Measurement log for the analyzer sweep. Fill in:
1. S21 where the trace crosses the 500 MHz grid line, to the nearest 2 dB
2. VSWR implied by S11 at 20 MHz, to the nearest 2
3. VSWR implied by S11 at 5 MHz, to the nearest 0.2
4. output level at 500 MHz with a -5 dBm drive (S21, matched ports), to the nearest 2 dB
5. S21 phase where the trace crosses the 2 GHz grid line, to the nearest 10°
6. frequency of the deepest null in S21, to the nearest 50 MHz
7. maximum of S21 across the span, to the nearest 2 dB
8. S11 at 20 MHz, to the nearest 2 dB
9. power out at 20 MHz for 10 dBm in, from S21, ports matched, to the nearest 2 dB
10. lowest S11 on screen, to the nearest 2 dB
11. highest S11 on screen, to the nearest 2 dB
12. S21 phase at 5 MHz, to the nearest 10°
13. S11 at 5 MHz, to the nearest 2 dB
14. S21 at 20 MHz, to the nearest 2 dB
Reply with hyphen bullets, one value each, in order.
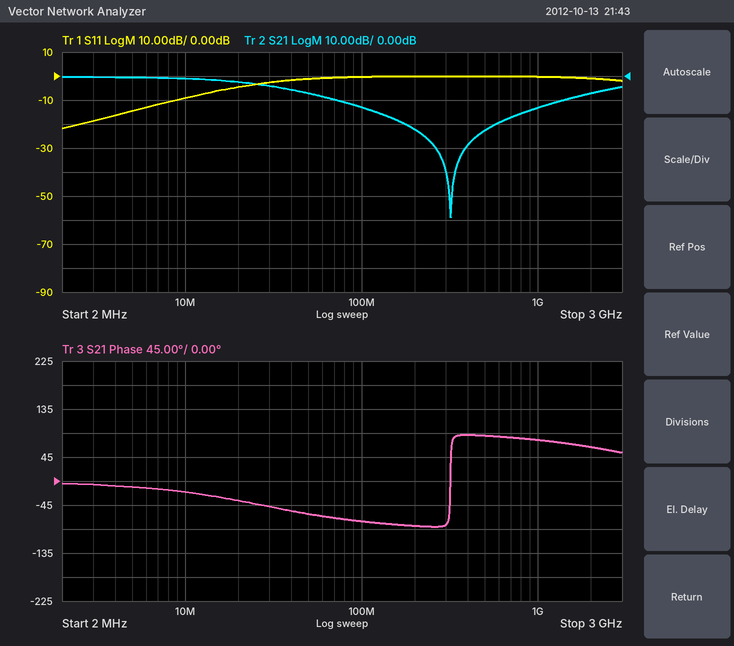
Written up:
- -22 dB
- 4
- 1.4
- -28 dBm
- 60°
- 300 MHz
- 0 dB
- -4 dB
- 8 dBm
- -22 dB
- 0 dB
- -10°
- -14 dB
- -2 dB
